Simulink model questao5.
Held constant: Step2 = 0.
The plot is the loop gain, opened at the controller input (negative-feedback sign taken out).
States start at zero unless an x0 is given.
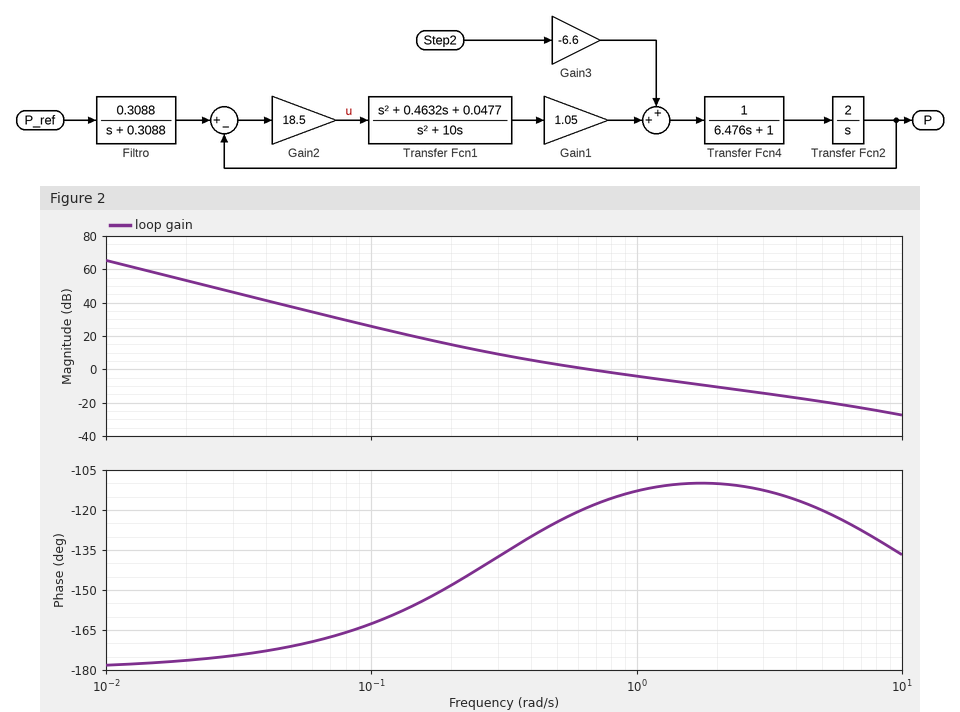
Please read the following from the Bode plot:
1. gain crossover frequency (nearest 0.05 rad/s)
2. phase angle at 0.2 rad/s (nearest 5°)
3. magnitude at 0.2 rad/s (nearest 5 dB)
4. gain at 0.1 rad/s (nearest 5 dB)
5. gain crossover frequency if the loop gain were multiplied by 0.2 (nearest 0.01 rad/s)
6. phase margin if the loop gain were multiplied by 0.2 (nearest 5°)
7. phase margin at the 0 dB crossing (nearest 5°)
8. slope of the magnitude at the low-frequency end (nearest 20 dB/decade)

0.65 rad/s
-150°
15 dB
25 dB
0.21 rad/s
35°
60°
-40 dB/decade
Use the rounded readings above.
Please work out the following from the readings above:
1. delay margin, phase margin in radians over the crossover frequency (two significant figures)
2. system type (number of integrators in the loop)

1.6 s
2
